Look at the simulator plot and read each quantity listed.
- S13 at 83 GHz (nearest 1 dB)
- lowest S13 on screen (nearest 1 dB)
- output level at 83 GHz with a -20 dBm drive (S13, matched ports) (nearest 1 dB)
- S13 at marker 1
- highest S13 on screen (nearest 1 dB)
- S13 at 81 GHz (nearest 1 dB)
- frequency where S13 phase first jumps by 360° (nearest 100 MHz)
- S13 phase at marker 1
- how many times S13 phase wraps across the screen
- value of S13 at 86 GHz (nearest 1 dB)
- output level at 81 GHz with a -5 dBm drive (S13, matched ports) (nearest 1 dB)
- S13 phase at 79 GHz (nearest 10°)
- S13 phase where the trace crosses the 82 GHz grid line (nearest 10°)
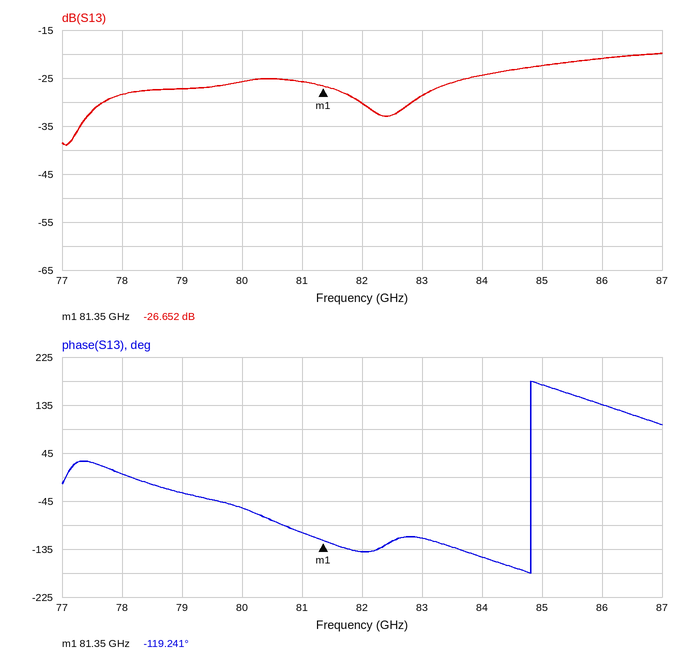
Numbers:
-29 dB
-39 dB
-49 dBm
-26.652 dB
-20 dB
-26 dB
84.8 GHz
-119.241°
1
-21 dB
-31 dBm
-30°
-140°
